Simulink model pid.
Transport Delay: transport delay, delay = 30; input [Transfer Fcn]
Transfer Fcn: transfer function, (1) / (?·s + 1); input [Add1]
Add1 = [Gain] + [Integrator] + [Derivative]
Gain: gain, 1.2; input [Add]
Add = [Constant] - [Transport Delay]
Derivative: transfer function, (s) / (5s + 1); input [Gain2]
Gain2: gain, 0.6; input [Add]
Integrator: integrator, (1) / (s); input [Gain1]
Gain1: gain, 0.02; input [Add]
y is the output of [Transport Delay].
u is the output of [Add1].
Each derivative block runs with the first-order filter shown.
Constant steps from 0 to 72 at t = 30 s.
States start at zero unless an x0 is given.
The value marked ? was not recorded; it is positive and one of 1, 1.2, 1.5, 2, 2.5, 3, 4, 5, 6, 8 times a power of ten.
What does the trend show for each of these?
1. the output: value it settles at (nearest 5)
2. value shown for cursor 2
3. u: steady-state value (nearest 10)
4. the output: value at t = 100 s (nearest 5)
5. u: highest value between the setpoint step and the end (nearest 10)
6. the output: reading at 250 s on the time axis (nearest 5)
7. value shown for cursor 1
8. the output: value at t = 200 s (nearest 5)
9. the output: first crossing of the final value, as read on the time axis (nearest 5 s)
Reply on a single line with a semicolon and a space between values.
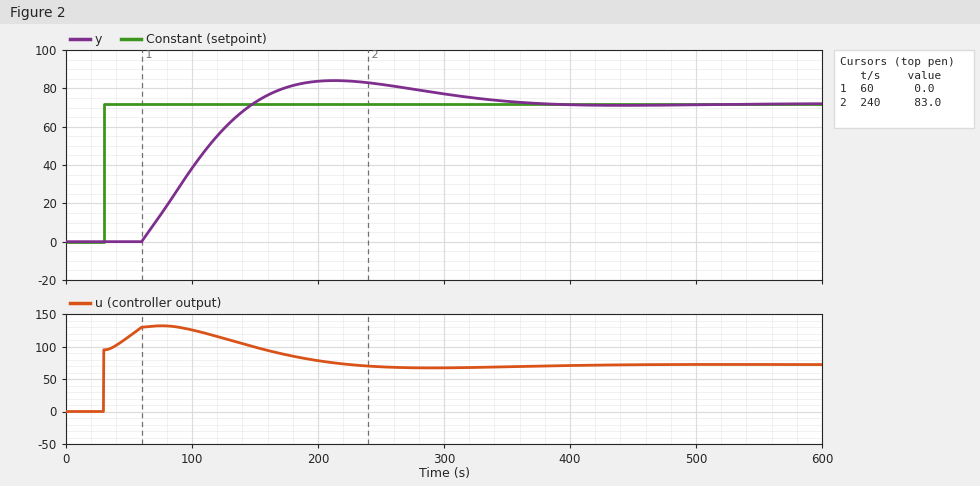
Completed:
70; 83.0; 70; 40; 130; 80; 0.0; 85; 150 s
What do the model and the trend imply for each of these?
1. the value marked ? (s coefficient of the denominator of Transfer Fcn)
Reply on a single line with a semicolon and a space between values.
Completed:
100
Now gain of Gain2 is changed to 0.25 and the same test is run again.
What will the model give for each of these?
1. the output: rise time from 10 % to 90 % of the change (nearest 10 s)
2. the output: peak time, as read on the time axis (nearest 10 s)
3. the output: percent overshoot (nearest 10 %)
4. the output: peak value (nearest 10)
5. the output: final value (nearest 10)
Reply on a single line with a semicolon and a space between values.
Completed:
70 s; 210 s; 20 %; 80; 70
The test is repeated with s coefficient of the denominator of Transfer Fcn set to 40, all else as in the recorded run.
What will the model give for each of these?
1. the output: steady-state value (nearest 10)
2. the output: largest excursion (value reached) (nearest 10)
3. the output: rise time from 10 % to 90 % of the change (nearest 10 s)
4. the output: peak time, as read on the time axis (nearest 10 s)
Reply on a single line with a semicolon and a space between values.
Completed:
70; 80; 30 s; 120 s
